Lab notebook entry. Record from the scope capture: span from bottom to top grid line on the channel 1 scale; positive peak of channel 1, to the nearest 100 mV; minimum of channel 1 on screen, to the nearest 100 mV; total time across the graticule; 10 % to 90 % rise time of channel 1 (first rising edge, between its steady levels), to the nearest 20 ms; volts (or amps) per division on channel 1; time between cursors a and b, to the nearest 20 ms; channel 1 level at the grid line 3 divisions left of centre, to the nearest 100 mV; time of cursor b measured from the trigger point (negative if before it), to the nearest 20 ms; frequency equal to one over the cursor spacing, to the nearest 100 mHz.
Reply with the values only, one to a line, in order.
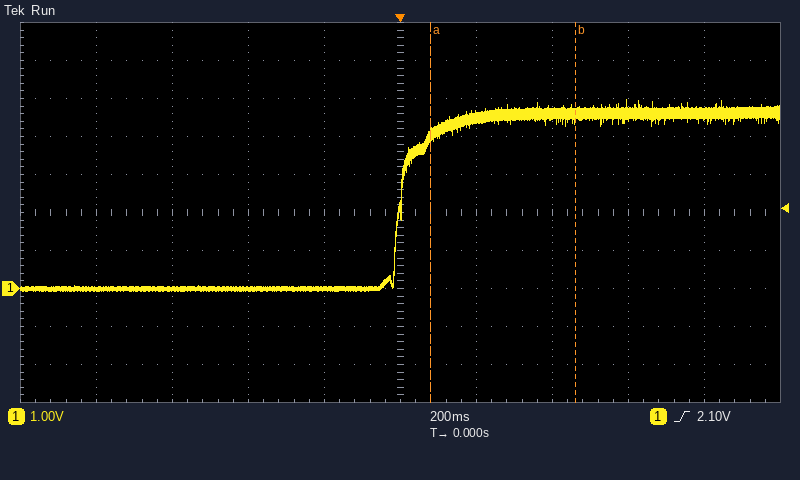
10 V
5.0 V
-100 mV
2 s
120 ms
1 V
380 ms
0.0 V
+460 ms
2.6 Hz
